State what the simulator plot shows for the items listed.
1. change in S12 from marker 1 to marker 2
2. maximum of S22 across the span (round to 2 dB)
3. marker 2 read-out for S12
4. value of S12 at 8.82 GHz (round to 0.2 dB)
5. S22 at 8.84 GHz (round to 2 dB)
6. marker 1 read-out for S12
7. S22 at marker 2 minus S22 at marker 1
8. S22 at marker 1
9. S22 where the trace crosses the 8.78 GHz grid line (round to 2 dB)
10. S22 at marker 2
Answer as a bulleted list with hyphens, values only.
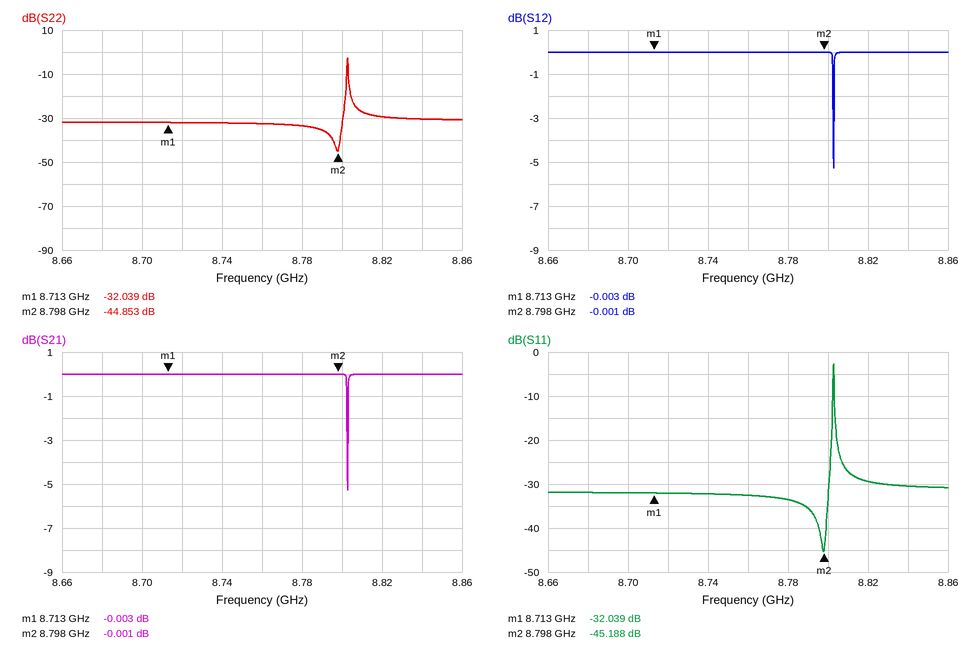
- 0.002 dB
- -2 dB
- -0.001 dB
- 0.0 dB
- -30 dB
- -0.003 dB
- -12.814 dB
- -32.039 dB
- -34 dB
- -44.853 dB
